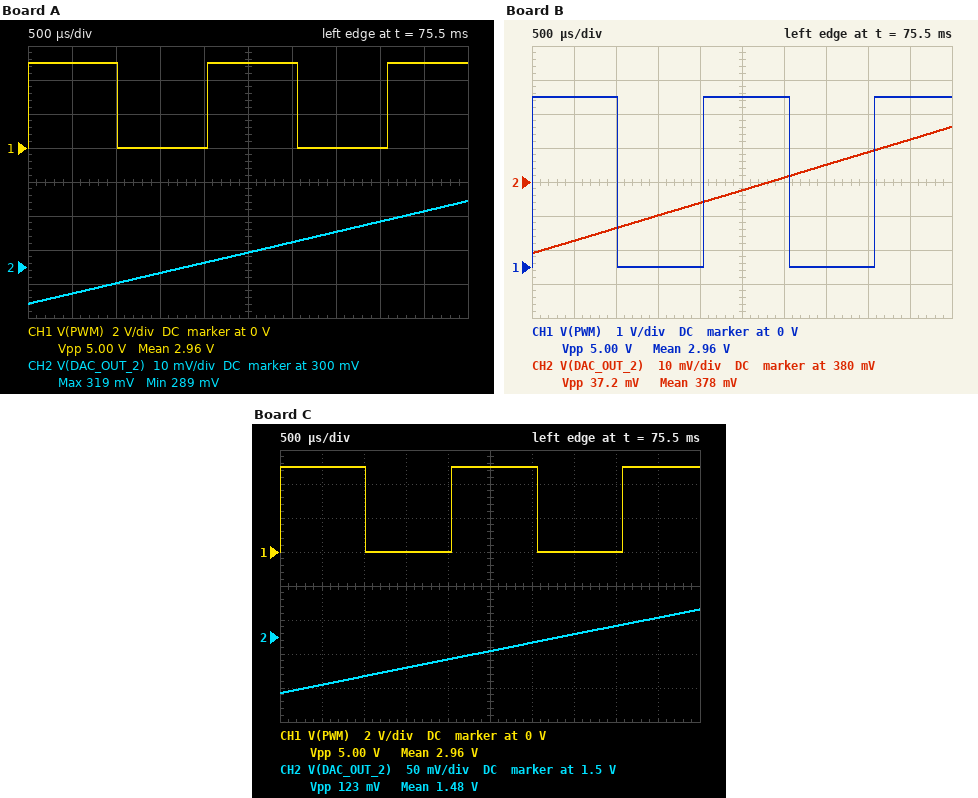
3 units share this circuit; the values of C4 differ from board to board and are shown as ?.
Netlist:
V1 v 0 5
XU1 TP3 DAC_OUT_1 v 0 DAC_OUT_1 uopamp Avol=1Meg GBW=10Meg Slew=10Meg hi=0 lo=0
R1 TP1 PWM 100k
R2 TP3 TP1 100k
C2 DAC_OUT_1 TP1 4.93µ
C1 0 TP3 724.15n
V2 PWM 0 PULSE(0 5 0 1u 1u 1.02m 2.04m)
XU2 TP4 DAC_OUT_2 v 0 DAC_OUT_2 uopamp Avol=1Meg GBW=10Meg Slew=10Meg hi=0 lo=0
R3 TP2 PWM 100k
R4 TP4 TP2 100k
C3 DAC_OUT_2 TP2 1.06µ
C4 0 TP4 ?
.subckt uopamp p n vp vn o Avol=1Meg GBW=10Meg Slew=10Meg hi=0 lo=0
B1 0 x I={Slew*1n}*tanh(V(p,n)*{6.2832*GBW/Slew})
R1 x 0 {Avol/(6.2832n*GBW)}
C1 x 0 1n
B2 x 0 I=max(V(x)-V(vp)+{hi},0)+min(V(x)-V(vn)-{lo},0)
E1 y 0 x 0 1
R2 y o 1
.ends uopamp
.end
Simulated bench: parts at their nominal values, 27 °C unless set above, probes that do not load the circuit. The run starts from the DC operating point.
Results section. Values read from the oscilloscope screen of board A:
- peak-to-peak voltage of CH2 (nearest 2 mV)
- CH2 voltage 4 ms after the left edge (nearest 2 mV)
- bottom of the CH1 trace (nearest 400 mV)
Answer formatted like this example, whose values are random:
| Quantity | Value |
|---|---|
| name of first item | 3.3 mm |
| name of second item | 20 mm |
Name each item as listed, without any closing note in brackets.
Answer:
| Quantity | Value |
|---|---|
| peak-to-peak voltage of CH2 | 30 mV |
| CH2 voltage 4 ms after the left edge | 314 mV |
| bottom of the CH1 trace | 0 V |
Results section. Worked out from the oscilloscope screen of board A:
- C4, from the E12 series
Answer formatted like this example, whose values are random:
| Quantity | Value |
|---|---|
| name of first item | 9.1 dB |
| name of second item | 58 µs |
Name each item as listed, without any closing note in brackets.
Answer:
| Quantity | Value |
|---|---|
| C4, from the E12 series | 1.5 µF |
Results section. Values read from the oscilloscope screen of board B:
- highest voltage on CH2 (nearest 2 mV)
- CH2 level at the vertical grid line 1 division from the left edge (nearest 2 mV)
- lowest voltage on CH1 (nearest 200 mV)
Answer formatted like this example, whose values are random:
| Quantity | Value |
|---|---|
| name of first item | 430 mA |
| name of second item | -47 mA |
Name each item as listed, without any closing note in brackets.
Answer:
| Quantity | Value |
|---|---|
| highest voltage on CH2 | 396 mV |
| CH2 level at the vertical grid line 1 division from the left edge | 362 mV |
| lowest voltage on CH1 | 0 V |
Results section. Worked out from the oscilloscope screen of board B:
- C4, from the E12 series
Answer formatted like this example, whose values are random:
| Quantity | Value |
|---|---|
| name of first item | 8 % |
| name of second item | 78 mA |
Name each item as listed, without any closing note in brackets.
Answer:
| Quantity | Value |
|---|---|
| C4, from the E12 series | 1.2 µF |
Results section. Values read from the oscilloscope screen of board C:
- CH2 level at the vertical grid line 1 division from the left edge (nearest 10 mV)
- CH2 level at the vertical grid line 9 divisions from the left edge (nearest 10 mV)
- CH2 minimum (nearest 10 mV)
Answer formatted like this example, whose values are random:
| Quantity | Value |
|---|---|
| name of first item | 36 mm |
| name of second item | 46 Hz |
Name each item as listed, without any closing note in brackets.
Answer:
| Quantity | Value |
|---|---|
| CH2 level at the vertical grid line 1 division from the left edge | 1.43 V |
| CH2 level at the vertical grid line 9 divisions from the left edge | 1.53 V |
| CH2 minimum | 1.42 V |
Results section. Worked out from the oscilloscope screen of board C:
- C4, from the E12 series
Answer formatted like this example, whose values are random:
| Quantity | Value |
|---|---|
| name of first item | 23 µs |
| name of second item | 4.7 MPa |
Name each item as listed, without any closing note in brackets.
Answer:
| Quantity | Value |
|---|---|
| C4, from the E12 series | 270 nF |
